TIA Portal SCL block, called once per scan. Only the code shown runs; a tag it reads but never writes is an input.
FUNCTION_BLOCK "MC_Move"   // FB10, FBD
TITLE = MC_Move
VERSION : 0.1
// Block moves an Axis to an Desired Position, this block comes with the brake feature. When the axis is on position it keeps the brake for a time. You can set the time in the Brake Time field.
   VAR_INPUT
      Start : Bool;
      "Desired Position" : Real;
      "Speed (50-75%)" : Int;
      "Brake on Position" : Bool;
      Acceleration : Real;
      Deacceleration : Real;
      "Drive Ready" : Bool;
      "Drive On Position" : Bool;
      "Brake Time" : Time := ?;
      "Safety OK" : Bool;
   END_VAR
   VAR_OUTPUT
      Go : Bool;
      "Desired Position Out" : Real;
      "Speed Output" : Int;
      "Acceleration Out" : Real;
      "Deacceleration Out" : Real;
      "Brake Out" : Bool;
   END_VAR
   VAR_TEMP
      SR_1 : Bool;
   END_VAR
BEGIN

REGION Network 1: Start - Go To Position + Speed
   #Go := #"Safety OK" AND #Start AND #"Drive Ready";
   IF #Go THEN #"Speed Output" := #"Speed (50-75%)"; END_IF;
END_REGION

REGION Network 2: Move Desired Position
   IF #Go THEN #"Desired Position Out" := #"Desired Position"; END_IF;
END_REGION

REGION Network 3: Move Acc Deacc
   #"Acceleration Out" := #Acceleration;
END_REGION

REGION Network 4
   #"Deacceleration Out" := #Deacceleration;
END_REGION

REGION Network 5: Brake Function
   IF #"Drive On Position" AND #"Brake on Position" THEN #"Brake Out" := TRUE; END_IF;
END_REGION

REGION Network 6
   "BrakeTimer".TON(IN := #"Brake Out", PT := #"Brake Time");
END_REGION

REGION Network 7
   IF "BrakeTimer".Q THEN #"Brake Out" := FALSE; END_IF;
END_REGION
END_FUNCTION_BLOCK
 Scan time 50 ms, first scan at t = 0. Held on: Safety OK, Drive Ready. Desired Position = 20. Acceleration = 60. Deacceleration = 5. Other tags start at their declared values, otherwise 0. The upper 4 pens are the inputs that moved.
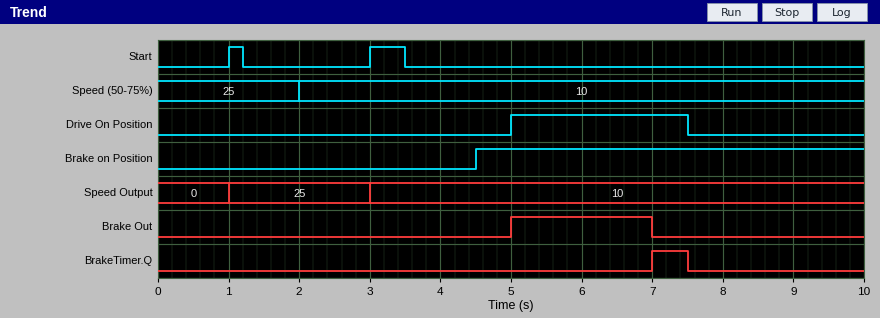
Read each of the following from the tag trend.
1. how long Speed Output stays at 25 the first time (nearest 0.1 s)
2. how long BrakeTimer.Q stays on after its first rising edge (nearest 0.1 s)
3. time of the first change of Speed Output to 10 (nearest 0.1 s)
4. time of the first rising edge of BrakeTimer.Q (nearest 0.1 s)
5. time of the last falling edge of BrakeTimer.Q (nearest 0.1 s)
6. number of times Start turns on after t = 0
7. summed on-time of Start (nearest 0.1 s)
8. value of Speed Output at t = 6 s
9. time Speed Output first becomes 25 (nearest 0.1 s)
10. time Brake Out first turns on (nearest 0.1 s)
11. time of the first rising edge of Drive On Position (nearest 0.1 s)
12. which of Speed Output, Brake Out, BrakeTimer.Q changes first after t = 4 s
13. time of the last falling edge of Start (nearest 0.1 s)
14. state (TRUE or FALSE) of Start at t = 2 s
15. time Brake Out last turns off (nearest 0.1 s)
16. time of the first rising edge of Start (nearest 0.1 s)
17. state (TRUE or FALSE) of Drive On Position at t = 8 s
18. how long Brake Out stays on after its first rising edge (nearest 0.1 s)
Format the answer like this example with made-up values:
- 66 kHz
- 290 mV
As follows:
- 2.0 s
- 0.5 s
- 3.0 s
- 7.0 s
- 7.5 s
- 2
- 0.7 s
- 10
- 1.0 s
- 5.0 s
- 5.0 s
- Brake Out
- 3.5 s
- FALSE
- 7.0 s
- 1.0 s
- FALSE
- 2.0 s
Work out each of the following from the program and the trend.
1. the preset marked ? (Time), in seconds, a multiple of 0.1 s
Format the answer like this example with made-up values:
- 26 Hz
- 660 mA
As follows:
- 2.0 s
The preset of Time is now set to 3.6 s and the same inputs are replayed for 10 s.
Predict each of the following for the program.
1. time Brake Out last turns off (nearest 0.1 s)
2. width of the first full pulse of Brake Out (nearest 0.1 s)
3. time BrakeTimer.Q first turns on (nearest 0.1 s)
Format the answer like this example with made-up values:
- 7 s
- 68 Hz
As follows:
- 8.6 s
- 3.6 s
- 8.6 s
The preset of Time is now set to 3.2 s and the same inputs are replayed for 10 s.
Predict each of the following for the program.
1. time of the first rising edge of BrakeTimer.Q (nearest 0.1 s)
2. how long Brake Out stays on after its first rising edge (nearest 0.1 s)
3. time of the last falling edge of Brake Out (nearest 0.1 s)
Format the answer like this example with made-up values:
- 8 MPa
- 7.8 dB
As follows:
- 8.2 s
- 3.2 s
- 8.2 s
